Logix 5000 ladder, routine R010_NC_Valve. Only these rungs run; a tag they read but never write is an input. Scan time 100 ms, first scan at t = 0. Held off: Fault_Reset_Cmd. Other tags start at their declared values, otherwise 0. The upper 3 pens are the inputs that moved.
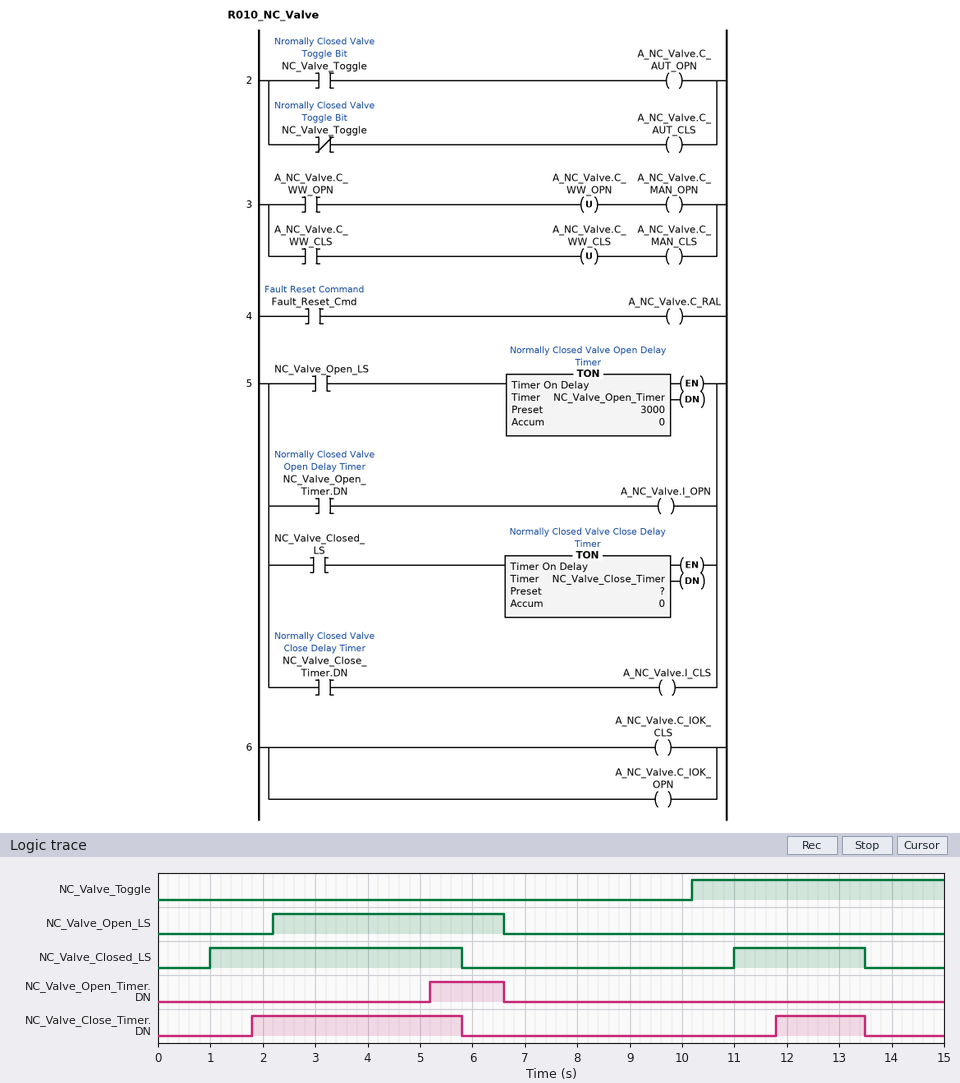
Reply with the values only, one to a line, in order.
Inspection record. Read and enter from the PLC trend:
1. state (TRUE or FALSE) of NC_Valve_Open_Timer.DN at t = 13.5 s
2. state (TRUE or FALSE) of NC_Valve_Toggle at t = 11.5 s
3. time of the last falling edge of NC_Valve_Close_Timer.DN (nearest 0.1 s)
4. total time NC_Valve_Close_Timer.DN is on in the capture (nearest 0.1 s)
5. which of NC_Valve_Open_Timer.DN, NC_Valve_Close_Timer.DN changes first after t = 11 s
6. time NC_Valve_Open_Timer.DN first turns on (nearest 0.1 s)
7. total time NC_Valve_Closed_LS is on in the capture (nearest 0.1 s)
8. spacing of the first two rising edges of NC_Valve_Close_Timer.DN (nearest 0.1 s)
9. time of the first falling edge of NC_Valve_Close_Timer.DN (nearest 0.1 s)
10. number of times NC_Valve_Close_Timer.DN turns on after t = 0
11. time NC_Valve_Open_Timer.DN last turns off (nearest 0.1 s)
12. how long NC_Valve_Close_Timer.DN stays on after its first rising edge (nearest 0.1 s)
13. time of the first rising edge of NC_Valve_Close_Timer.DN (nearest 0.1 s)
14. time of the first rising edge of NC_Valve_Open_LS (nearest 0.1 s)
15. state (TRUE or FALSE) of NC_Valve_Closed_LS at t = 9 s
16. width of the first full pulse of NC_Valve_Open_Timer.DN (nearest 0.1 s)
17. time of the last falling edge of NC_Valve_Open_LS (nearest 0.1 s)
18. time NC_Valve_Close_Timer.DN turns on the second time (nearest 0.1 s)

FALSE
TRUE
13.5 s
5.7 s
NC_Valve_Close_Timer.DN
5.2 s
7.3 s
10.0 s
5.8 s
2
6.6 s
4.0 s
1.8 s
2.2 s
FALSE
1.4 s
6.6 s
11.8 s
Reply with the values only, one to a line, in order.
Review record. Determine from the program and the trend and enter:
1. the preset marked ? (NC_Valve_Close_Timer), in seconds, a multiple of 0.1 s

0.8 s
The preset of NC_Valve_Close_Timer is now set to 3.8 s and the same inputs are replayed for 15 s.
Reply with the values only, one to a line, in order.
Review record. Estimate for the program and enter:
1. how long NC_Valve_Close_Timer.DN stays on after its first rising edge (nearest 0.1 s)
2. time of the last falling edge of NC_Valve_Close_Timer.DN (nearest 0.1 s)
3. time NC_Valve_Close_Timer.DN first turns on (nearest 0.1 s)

1.0 s
5.8 s
4.8 s
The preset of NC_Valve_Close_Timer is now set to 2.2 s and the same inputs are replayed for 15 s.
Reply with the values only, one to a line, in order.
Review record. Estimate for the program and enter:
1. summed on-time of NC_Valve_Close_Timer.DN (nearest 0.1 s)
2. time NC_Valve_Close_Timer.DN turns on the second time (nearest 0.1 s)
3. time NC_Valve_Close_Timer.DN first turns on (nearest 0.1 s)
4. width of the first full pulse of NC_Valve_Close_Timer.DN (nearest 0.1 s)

2.9 s
13.2 s
3.2 s
2.6 s
